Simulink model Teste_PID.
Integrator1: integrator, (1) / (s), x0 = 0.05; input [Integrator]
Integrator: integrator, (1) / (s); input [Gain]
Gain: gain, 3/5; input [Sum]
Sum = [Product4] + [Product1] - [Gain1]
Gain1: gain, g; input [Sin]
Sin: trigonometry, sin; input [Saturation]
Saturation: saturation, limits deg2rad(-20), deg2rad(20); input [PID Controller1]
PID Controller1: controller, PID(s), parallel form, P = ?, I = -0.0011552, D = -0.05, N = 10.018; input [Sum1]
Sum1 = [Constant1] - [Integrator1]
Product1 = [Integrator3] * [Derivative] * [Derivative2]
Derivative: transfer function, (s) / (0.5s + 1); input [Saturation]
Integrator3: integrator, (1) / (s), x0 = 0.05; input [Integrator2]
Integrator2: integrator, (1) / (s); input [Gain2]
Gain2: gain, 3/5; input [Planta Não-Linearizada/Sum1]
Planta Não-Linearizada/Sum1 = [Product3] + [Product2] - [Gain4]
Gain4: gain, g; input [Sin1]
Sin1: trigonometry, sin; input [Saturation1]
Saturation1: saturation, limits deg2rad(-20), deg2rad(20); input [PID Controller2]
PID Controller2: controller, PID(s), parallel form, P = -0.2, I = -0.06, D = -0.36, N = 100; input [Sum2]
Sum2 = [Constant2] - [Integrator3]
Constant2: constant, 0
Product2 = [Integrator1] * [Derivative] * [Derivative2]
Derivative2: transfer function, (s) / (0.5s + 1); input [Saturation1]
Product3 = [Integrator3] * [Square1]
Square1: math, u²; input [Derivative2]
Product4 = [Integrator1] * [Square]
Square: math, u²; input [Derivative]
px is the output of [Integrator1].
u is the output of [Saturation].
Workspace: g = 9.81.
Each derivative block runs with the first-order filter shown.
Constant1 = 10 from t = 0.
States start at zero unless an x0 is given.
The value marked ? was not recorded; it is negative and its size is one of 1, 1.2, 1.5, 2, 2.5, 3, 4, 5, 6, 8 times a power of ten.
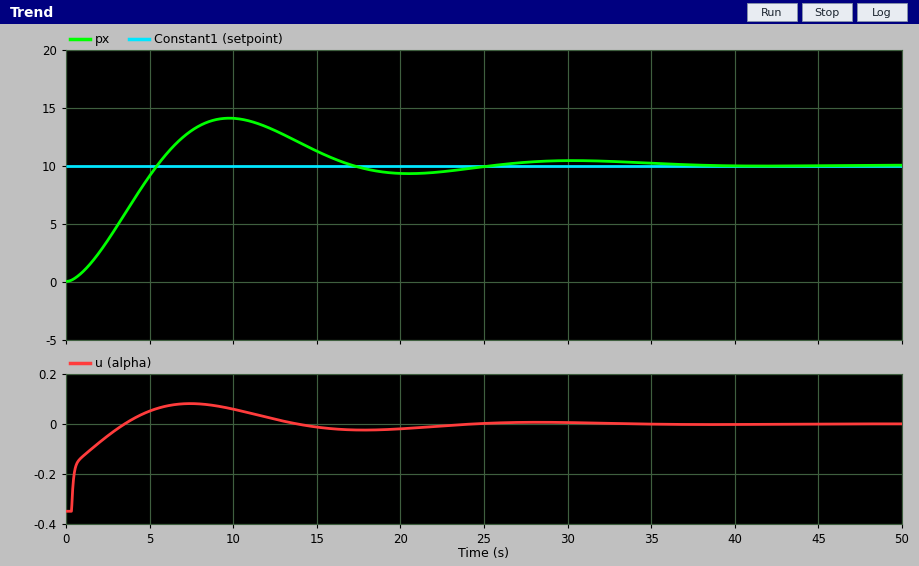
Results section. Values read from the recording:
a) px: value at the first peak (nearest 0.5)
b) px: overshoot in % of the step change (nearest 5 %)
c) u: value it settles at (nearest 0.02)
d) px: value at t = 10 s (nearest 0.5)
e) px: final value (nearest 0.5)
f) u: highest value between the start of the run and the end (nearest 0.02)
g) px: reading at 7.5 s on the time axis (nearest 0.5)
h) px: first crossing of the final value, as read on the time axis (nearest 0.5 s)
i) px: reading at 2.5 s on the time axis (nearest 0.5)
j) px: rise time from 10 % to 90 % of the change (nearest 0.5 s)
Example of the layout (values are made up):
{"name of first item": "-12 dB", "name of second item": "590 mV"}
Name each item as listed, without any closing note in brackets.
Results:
{"px: value at the first peak": "14.0", "px: overshoot in % of the step change": "40 %", "u: value it settles at": "0.00", "px: value at t = 10 s": "14.0", "px: final value": "10.0", "u: highest value between the start of the run and the end": "0.08", "px: reading at 7.5 s on the time axis": "13.0", "px: first crossing of the final value, as read on the time axis": "5.5 s", "px: reading at 2.5 s on the time axis": "3.5", "px: rise time from 10 % to 90 % of the change": "4.0 s"}
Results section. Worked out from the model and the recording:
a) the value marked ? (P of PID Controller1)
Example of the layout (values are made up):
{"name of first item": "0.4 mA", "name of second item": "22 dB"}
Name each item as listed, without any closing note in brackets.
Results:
{"the value marked ?": "-0.02"}
